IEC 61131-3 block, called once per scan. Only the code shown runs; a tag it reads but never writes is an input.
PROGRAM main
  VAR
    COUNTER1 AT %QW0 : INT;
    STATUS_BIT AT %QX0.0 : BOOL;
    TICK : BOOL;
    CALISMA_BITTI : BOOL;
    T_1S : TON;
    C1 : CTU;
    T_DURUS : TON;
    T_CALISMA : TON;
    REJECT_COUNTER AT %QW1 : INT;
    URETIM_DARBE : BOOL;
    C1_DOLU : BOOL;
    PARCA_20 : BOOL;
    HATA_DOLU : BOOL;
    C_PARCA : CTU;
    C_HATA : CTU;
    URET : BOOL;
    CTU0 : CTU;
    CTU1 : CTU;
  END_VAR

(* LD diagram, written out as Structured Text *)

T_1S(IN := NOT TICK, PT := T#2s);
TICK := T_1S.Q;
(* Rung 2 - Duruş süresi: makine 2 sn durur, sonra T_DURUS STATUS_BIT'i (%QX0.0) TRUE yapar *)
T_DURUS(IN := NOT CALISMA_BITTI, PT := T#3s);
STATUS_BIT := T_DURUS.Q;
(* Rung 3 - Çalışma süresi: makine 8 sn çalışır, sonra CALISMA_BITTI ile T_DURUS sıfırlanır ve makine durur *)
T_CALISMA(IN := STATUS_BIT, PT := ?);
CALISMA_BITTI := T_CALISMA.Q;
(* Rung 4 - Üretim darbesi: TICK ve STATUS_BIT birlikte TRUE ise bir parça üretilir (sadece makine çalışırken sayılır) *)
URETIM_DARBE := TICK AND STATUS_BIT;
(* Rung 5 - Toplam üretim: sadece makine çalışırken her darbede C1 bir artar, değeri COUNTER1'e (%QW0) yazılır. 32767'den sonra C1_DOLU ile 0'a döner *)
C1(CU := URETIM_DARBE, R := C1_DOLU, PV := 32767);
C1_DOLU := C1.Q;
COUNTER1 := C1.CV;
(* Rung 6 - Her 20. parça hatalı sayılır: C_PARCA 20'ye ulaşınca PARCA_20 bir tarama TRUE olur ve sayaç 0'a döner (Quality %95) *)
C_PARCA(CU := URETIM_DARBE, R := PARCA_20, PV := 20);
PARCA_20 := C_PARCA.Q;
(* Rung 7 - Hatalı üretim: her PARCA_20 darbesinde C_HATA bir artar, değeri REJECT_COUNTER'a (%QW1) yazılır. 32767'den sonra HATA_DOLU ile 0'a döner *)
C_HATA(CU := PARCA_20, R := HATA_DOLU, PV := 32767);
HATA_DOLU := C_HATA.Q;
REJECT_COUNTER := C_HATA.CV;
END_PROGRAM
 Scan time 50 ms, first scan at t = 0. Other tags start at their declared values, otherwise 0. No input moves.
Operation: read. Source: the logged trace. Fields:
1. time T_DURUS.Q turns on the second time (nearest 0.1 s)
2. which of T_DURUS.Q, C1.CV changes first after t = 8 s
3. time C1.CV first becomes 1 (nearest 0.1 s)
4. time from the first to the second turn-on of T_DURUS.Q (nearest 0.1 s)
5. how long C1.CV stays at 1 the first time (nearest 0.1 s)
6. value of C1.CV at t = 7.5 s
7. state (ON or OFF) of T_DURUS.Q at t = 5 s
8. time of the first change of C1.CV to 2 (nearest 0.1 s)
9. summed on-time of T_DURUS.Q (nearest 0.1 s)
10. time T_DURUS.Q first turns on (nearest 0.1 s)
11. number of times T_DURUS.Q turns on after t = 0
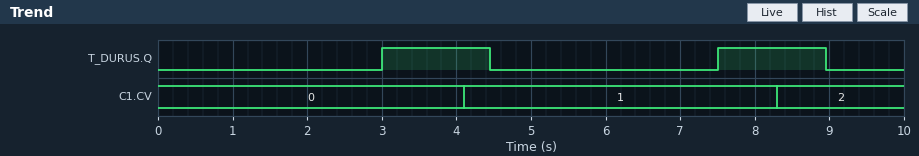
7.5 s
C1.CV
4.1 s
4.5 s
4.2 s
1
OFF
8.3 s
2.9 s
3.0 s
2
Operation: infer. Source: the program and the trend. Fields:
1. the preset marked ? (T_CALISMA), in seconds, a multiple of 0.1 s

1.4 s
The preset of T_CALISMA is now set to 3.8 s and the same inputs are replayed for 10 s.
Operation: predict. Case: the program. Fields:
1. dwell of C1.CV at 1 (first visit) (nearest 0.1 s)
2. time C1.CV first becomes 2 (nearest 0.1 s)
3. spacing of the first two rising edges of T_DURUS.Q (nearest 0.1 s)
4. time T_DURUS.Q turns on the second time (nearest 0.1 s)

2.1 s
6.2 s
6.9 s
9.9 s
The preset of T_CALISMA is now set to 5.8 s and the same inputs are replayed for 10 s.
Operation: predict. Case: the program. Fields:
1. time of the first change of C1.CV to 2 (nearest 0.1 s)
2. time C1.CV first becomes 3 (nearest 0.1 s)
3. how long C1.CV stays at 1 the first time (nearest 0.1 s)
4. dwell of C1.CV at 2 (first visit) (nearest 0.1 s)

6.2 s
8.3 s
2.1 s
2.1 s
